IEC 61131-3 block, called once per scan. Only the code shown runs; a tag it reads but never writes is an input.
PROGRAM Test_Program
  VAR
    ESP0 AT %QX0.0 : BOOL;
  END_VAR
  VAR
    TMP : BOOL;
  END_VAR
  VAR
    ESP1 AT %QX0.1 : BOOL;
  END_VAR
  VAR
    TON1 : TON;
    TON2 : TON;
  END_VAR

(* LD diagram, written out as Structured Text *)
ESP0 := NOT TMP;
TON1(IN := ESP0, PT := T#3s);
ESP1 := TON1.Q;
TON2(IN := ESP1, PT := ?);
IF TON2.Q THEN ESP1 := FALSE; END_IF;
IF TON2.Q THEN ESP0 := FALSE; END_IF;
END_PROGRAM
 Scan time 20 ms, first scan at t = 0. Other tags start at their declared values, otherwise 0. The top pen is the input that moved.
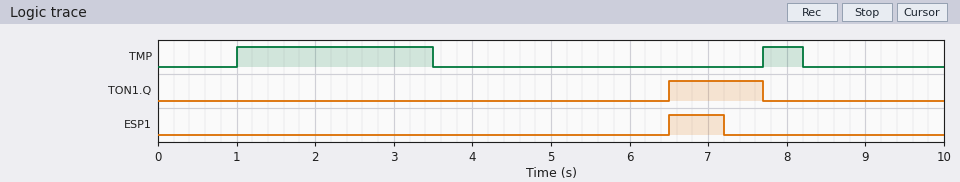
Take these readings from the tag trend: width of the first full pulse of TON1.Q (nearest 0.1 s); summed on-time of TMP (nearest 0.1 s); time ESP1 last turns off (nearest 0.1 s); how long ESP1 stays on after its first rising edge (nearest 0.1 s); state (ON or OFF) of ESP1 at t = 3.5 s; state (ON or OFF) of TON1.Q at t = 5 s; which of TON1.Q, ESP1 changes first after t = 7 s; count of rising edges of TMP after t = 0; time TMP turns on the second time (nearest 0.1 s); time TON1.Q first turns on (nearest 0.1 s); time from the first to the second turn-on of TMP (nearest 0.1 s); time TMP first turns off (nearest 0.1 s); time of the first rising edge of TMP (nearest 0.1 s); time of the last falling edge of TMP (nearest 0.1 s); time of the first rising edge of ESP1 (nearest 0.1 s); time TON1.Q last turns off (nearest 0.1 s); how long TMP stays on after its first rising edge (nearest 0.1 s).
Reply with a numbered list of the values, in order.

1. 1.2 s
2. 3.0 s
3. 7.2 s
4. 0.7 s
5. OFF
6. OFF
7. ESP1
8. 2
9. 7.7 s
10. 6.5 s
11. 6.7 s
12. 3.5 s
13. 1.0 s
14. 8.2 s
15. 6.5 s
16. 7.7 s
17. 2.5 s
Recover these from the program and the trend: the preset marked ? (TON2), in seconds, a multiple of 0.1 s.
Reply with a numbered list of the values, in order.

1. 0.7 s
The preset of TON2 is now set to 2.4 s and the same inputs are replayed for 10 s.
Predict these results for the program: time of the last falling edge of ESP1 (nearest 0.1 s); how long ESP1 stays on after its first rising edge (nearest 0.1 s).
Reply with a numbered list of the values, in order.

1. 7.7 s
2. 1.2 s
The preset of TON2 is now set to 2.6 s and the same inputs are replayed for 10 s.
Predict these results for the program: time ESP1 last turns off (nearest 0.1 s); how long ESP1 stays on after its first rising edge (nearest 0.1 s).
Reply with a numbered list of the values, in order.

1. 7.7 s
2. 1.2 s
